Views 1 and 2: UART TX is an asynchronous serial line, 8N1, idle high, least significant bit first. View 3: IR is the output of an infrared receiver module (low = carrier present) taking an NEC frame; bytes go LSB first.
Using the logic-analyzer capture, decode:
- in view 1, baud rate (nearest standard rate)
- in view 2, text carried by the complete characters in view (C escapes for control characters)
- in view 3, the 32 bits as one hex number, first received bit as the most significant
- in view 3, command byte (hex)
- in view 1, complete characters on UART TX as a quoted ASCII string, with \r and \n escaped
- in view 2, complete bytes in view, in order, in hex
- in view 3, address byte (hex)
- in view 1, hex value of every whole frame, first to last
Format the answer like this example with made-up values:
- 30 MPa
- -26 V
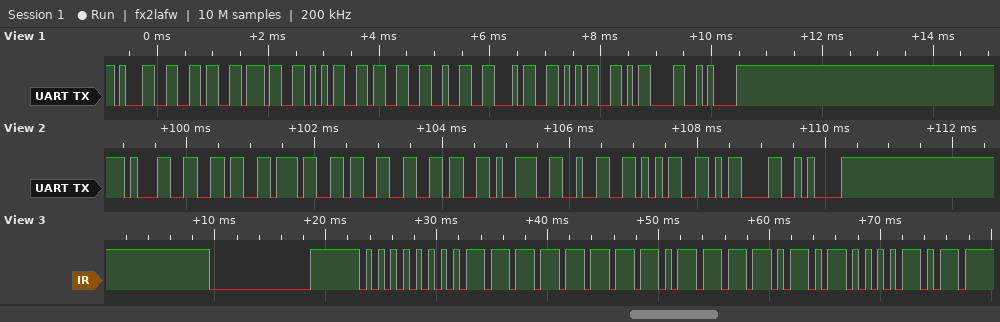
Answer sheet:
- 9600 baud
- "16736925\r\n"
- 0x00FF7A85
- 0x5E
- "16753245\r\n"
- 0x31 0x36 0x37 0x33 0x36 0x39 0x32 0x35 0x0D 0x0A
- 0x00
- 31 36 37 35 33 32 34 35 0D 0A
